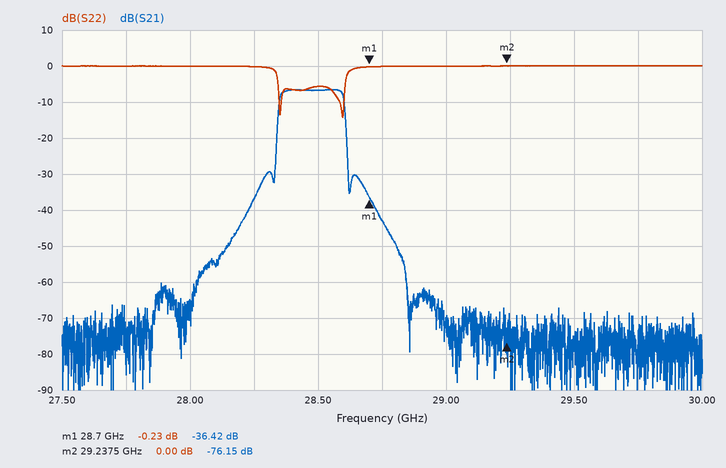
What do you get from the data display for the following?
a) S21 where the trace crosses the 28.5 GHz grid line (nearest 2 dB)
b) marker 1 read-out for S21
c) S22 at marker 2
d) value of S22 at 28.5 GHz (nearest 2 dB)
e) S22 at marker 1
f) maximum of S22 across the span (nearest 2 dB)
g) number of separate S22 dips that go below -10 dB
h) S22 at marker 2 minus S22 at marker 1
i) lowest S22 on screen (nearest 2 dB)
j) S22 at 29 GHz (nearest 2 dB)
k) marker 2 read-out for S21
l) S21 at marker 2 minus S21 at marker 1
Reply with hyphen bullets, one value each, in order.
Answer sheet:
- -6 dB
- -36.42 dB
- 0.00 dB
- -6 dB
- -0.23 dB
- 0 dB
- 2
- 0.23 dB
- -14 dB
- 0 dB
- -76.15 dB
- -39.73 dB
